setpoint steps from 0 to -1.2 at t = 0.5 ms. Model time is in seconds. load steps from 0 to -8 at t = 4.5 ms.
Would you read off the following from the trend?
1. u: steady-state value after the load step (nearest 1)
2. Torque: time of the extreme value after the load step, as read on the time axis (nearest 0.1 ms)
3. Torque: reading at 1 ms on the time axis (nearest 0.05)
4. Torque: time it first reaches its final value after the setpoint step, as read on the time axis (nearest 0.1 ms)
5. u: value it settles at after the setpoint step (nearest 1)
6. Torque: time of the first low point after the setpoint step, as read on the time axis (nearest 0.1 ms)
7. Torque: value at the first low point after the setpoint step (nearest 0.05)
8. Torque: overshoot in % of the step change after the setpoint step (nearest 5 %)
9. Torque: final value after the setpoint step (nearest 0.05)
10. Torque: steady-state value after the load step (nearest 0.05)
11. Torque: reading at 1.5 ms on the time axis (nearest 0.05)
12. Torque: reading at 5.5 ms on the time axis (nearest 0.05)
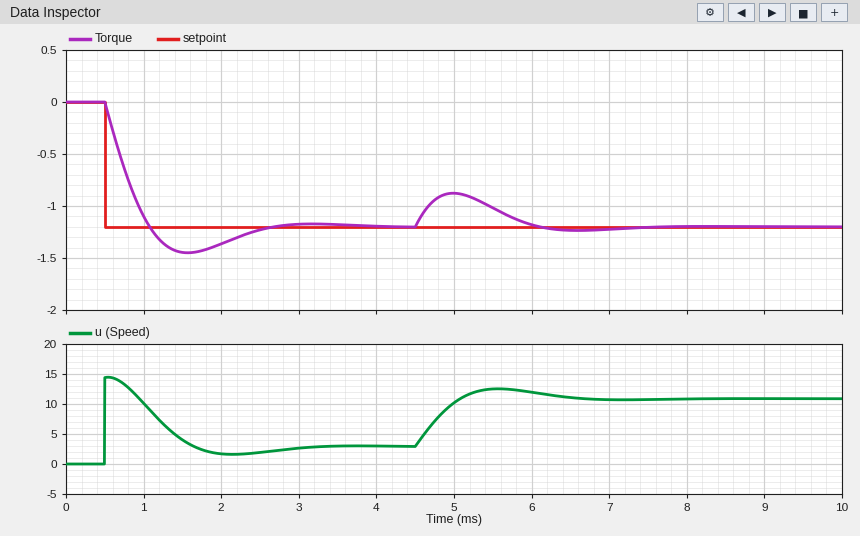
11
5.0 ms
-1.10
1.1 ms
3
1.6 ms
-1.45
20 %
-1.20
-1.20
-1.45
-1.00
